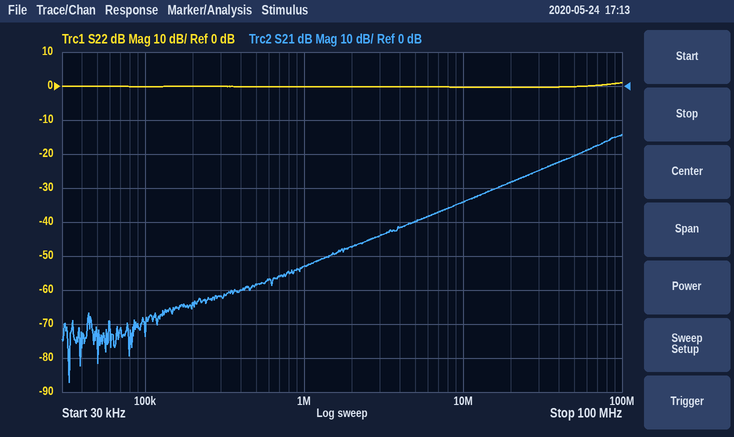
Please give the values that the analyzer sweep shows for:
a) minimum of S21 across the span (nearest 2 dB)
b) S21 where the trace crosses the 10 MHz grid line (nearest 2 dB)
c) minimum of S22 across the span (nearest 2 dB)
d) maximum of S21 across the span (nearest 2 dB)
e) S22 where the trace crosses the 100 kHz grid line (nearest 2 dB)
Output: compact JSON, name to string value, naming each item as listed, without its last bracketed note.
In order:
{"minimum of S21 across the span": "-88 dB", "S21 where the trace crosses the 10 MHz grid line": "-34 dB", "minimum of S22 across the span": "0 dB", "maximum of S21 across the span": "-14 dB", "S22 where the trace crosses the 100 kHz grid line": "0 dB"}
